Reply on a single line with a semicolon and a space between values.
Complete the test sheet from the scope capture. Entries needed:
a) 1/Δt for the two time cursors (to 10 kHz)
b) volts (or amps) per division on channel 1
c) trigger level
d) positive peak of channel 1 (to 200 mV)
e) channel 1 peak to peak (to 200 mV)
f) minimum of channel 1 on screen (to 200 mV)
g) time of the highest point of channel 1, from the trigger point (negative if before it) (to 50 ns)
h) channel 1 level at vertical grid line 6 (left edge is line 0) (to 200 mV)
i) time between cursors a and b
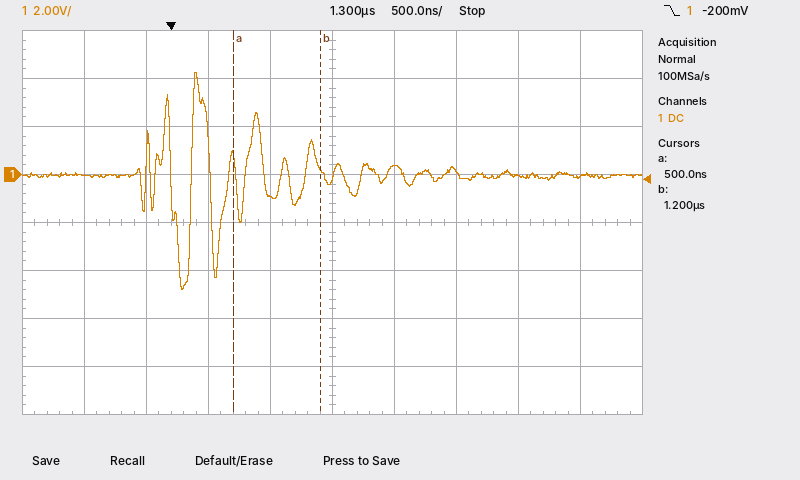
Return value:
1.43 MHz; 2 V; -200 mV; 4.2 V; 9.0 V; -4.8 V; +200 ns; 400 mV; 700 ns
